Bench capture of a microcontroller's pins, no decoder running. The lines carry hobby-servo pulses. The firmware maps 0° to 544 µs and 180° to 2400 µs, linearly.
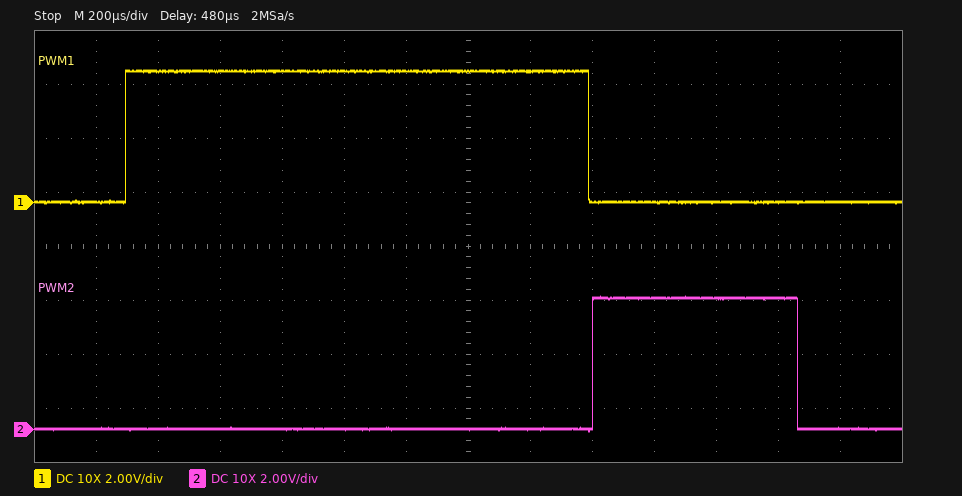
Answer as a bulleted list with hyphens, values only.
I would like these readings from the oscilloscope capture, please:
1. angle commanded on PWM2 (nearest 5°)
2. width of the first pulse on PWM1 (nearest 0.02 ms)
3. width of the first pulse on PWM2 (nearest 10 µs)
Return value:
- 10°
- 1.50 ms
- 660 µs
